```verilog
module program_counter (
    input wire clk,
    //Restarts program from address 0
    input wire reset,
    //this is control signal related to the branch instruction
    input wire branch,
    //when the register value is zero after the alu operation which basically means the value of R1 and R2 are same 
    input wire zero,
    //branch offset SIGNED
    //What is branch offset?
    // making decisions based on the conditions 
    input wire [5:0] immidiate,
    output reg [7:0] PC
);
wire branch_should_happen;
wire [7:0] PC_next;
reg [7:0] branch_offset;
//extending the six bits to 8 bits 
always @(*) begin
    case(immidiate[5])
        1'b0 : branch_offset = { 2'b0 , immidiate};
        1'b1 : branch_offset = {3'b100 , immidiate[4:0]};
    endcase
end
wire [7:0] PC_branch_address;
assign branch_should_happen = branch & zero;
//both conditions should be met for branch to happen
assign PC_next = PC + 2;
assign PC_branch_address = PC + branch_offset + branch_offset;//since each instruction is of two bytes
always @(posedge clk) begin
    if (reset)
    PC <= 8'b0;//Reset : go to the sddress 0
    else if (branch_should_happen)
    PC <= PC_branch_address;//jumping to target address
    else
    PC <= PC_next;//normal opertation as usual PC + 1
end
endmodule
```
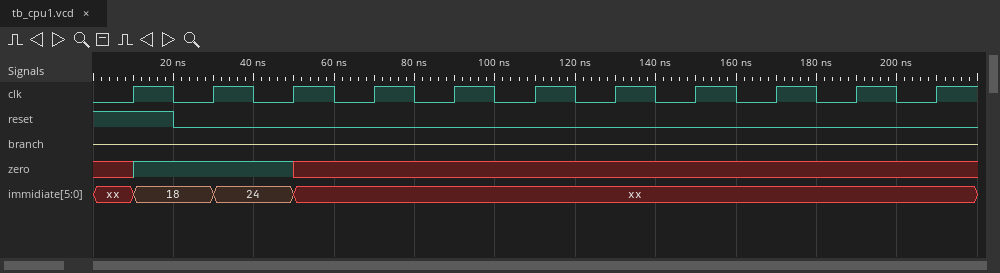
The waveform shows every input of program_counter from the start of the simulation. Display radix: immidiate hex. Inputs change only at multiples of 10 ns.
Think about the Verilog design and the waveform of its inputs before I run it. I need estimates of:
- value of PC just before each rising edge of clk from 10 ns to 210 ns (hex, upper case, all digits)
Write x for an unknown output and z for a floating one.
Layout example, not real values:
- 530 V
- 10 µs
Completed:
- x, 00, 02, 04, 06, 08, 0A, 0C, 0E, 10, 12
